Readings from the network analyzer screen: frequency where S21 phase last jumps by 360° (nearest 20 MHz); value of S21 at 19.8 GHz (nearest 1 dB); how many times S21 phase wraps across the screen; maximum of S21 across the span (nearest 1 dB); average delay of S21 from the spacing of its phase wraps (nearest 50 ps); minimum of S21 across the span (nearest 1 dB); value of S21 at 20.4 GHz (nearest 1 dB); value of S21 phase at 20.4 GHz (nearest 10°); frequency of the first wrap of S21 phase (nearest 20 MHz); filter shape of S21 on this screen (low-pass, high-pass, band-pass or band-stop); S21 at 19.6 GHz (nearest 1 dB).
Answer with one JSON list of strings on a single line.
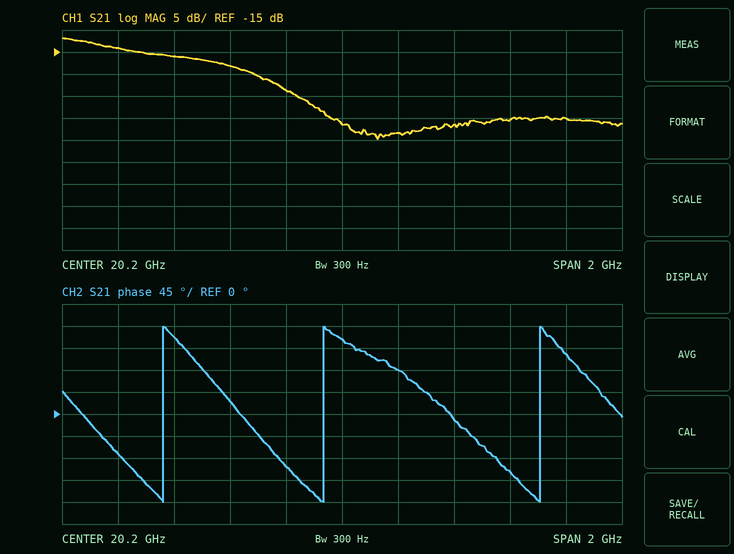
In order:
["20.90 GHz", "-18 dB", "3", "-12 dB", "1.50 ns", "-35 dB", "-33 dB", "90°", "19.56 GHz", "low-pass", "-16 dB"]
